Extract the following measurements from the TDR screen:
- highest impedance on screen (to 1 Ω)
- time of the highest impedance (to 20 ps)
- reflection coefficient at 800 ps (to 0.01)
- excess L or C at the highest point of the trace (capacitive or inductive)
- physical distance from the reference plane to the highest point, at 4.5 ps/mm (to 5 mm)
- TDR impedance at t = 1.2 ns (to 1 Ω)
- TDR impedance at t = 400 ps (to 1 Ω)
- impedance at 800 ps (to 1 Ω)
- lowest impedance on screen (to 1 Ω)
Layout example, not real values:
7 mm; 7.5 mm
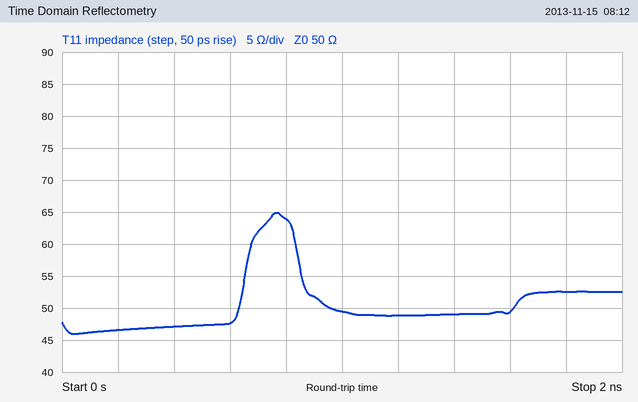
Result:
65 Ω; 760 ps; +0.12; inductive; 85 mm; 49 Ω; 47 Ω; 64 Ω; 46 Ω
